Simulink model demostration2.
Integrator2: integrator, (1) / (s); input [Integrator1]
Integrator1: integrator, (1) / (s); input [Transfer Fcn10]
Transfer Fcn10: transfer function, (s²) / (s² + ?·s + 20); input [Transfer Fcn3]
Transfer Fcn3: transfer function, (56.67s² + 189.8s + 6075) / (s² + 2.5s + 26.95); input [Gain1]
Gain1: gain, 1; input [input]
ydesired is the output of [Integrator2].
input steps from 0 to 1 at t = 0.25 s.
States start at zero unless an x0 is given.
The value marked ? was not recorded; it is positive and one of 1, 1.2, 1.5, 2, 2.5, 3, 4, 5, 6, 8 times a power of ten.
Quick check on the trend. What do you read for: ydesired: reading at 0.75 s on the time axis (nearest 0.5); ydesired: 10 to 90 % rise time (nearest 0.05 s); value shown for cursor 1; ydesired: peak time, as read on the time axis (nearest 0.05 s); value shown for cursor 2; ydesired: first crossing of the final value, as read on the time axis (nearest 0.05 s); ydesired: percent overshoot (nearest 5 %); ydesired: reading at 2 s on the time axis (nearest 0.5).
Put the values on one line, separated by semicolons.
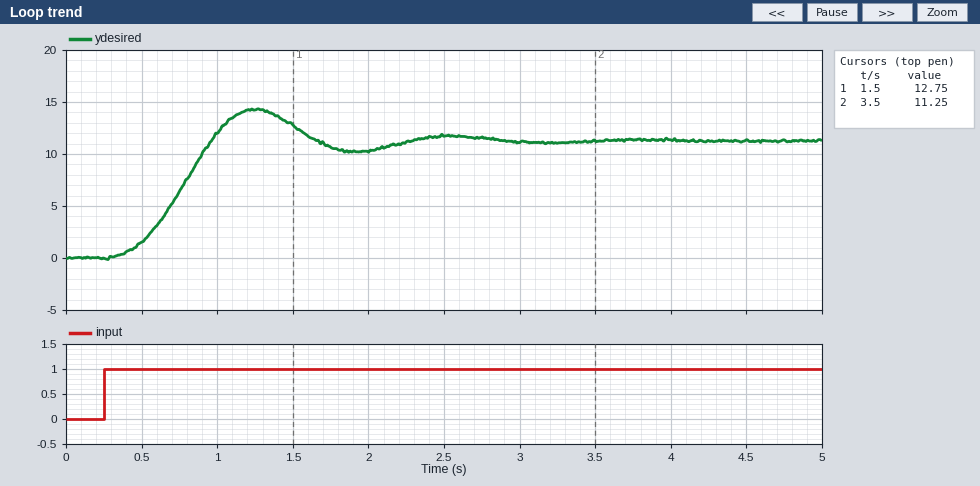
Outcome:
6.5; 0.45 s; 12.75; 1.25 s; 11.25; 0.95 s; 25 %; 10.5
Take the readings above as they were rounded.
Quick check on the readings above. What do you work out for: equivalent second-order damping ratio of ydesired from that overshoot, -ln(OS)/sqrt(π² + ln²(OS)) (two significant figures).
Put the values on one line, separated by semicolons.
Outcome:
0.40
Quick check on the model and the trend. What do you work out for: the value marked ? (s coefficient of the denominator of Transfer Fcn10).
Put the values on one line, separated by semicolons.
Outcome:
6
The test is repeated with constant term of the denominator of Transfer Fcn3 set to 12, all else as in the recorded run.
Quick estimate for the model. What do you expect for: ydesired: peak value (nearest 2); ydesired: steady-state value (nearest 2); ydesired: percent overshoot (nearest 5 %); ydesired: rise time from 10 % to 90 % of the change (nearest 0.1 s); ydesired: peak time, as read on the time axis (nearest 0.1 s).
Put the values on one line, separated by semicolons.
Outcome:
32; 26; 25 %; 0.6 s; 1.6 s
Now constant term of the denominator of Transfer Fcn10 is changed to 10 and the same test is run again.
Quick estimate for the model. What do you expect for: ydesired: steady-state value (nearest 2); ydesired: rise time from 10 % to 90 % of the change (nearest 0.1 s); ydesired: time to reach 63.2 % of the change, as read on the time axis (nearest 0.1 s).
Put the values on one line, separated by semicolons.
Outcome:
22; 0.7 s; 1.0 s
